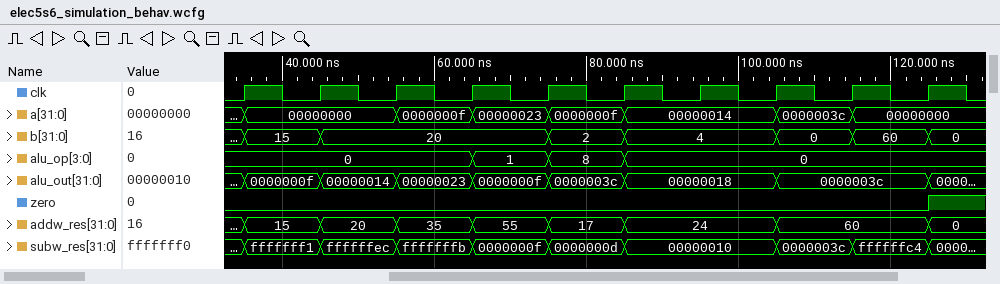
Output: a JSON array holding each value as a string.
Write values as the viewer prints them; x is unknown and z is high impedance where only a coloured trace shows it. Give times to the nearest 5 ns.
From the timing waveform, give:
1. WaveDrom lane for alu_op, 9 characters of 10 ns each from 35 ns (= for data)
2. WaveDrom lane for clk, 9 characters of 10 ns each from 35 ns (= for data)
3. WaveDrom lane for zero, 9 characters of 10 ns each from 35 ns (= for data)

["{name: 'alu_op', wave: '=..===...', data: '0 1 8 0'}", "{name: 'clk', wave: 'p........'}", "{name: 'zero', wave: '0........'}"]
